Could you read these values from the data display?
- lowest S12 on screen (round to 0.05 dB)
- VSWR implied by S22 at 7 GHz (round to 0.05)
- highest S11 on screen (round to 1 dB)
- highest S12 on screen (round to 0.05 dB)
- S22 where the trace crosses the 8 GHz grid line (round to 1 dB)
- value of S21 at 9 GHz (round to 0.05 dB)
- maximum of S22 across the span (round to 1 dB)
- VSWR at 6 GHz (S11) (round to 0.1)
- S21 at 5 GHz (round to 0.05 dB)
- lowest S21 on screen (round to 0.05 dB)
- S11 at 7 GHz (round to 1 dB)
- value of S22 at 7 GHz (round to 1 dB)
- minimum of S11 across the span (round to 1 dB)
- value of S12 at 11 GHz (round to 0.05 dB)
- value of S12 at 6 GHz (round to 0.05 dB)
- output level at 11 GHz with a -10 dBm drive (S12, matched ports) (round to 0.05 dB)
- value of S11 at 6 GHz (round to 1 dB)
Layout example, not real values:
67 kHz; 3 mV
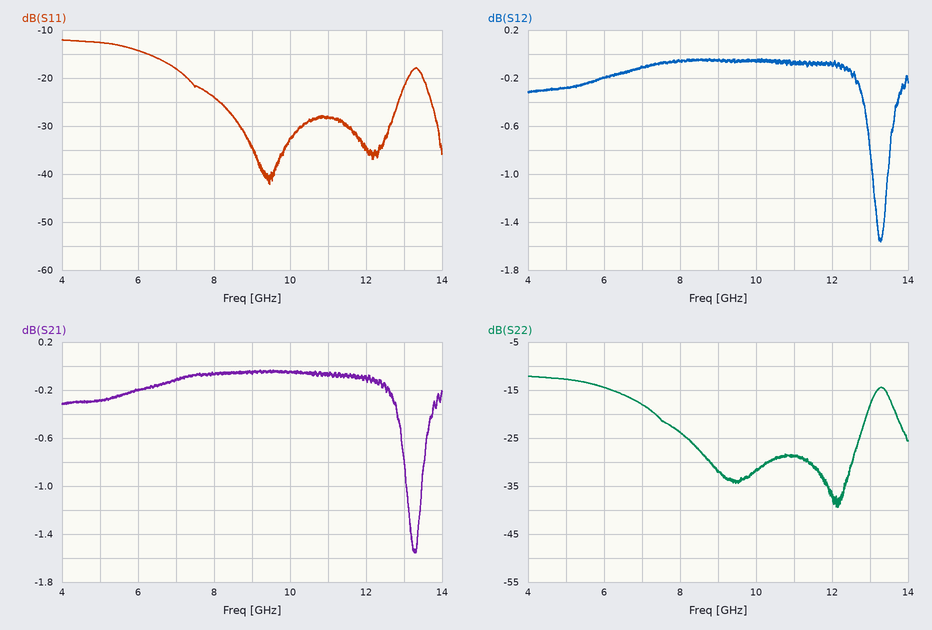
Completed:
-1.55 dB; 1.30; -12 dB; -0.05 dB; -24 dB; -0.05 dB; -12 dB; 1.5; -0.30 dB; -1.55 dB; -18 dB; -18 dB; -42 dB; -0.05 dB; -0.20 dB; -10.05 dBm; -14 dB
